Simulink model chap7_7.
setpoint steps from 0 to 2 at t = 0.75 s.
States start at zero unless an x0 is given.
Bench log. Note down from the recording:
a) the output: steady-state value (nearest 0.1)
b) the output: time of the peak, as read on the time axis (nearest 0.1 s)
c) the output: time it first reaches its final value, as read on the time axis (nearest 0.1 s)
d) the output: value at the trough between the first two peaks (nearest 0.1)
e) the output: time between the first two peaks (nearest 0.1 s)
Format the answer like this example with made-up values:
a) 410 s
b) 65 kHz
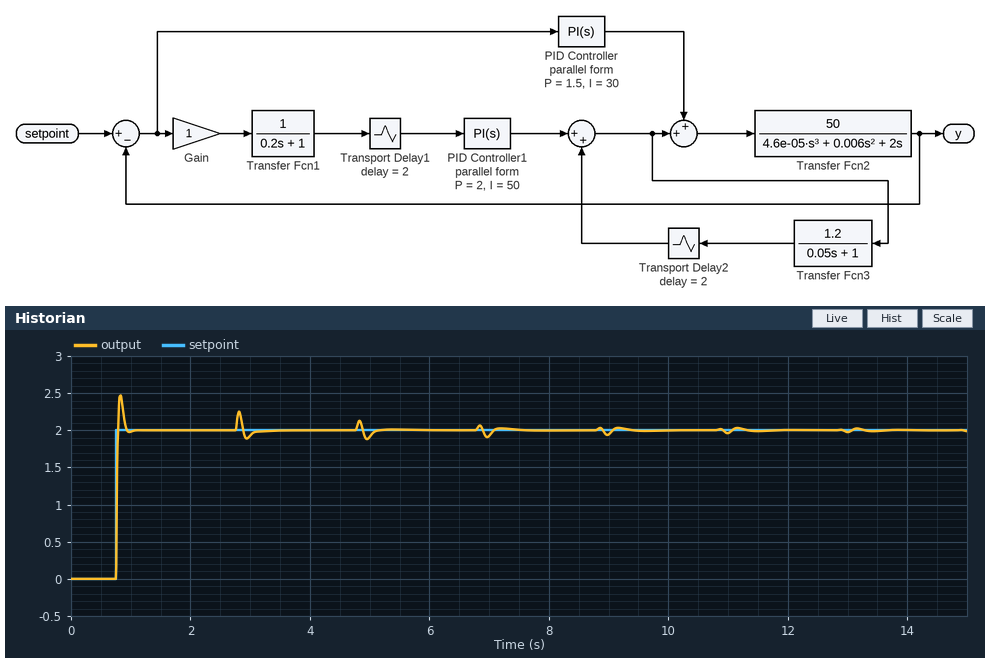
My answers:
a) 2.0
b) 0.8 s
c) 0.8 s
d) 2.0
e) 2.0 s
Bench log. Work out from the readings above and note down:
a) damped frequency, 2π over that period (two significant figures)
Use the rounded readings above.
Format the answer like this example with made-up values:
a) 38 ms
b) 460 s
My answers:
a) 3.1 rad/s
